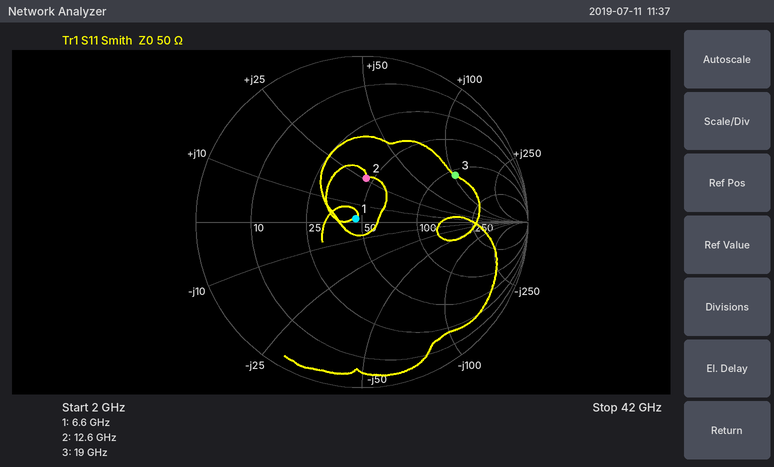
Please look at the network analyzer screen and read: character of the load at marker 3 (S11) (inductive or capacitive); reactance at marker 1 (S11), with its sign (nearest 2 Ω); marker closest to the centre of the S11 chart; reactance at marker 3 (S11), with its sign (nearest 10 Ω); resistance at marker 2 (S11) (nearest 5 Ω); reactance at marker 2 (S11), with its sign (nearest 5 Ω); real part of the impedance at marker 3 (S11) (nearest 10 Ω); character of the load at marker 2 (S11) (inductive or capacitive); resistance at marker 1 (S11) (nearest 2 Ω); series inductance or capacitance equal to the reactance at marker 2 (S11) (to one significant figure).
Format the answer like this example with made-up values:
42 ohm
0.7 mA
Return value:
inductive
+2 Ω
marker 1
+100 Ω
45 Ω
+25 Ω
110 Ω
inductive
46 Ω
300 pH
